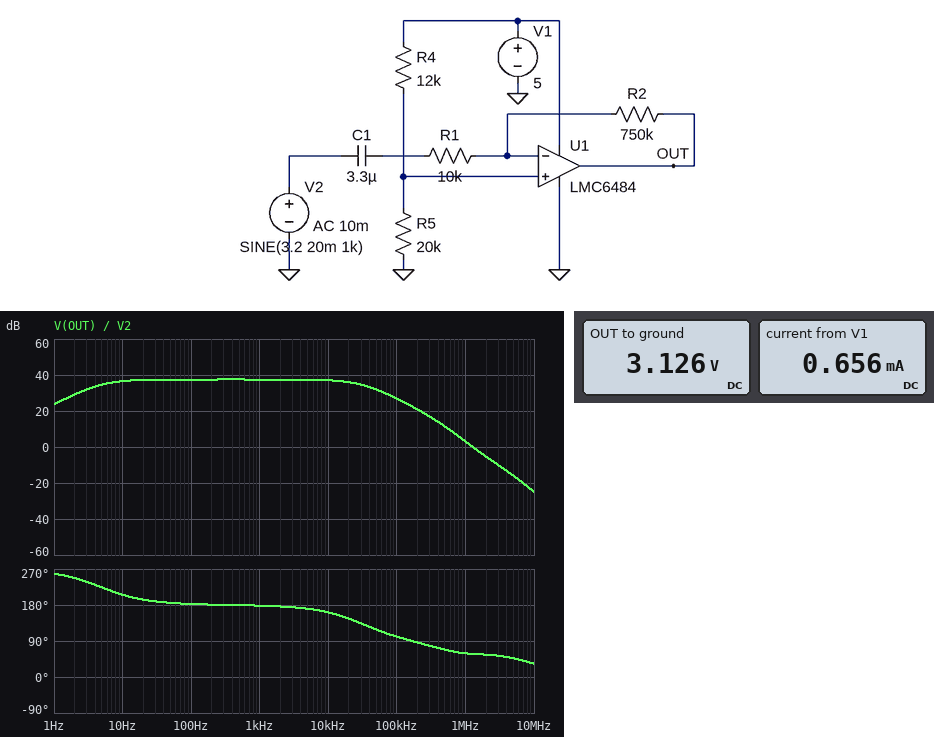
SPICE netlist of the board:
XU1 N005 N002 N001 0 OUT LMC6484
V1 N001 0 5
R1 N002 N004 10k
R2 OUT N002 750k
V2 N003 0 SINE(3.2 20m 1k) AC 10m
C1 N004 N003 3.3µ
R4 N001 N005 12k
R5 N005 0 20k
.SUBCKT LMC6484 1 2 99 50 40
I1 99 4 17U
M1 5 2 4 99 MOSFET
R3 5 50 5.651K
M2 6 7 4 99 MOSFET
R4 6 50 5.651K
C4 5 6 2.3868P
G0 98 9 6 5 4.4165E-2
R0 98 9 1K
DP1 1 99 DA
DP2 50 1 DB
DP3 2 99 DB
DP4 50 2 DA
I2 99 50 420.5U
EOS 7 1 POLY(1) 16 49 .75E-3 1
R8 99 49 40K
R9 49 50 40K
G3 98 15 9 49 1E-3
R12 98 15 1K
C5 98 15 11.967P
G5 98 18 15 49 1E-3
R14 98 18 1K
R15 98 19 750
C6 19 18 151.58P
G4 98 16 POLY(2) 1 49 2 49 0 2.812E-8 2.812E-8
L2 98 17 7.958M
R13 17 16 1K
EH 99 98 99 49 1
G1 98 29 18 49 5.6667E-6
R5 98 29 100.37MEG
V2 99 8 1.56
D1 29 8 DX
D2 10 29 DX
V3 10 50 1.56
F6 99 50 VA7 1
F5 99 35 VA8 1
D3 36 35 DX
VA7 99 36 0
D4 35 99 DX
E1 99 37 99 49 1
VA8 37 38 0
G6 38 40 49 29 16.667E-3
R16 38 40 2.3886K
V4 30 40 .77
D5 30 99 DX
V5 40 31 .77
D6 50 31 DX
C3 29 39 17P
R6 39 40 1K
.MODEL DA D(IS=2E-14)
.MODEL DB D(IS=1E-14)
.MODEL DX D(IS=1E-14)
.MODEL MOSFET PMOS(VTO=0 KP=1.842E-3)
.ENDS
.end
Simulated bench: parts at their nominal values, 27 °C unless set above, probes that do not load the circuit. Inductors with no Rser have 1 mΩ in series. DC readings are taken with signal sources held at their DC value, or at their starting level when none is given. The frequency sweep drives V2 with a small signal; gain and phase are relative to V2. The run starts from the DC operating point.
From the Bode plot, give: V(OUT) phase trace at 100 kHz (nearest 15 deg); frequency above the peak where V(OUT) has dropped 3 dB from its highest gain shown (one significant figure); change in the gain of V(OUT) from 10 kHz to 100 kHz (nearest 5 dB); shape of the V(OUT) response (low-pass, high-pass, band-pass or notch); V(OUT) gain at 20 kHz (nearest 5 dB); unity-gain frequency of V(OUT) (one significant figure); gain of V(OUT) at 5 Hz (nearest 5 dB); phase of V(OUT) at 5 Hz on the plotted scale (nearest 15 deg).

105 deg
30 kHz
-10 dB
band-pass
35 dB
1 MHz
35 dB
225 deg
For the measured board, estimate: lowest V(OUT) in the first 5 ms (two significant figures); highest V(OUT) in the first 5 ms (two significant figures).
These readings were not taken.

1.6 V
4.6 V
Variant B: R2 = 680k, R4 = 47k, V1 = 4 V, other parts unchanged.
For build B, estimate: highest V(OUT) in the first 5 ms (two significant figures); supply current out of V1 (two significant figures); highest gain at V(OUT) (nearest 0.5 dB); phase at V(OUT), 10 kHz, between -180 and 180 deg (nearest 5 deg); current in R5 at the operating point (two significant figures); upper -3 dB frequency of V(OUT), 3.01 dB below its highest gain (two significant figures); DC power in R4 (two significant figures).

2.6 V
550 µA
36.5 dB
165 deg
60 µA
34 kHz
170 µW
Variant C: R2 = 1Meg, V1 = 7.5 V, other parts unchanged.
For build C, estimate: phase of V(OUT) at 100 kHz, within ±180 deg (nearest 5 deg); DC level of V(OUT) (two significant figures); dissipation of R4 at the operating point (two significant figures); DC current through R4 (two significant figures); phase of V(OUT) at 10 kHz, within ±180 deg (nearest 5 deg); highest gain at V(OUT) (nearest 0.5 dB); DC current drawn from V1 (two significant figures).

95 deg
4.7 V
660 µW
230 µA
155 deg
40.0 dB
770 µA
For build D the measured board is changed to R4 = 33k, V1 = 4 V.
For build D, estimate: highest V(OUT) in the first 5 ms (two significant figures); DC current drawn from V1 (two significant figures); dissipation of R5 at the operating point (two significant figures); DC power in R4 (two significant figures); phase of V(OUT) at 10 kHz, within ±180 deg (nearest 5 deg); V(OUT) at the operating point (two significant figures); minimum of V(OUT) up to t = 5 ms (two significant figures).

3.0 V
560 µA
110 µW
190 µW
160 deg
1.5 V
55 mV
